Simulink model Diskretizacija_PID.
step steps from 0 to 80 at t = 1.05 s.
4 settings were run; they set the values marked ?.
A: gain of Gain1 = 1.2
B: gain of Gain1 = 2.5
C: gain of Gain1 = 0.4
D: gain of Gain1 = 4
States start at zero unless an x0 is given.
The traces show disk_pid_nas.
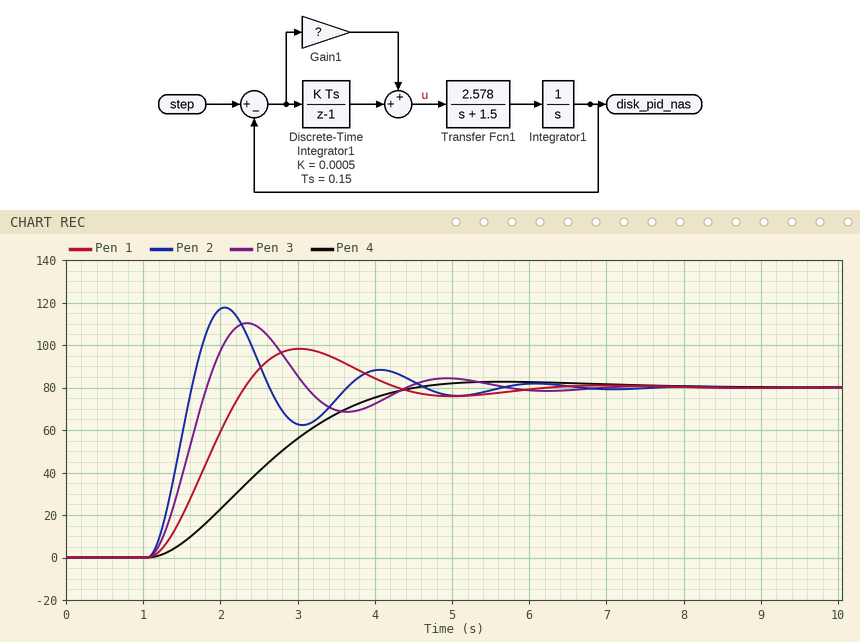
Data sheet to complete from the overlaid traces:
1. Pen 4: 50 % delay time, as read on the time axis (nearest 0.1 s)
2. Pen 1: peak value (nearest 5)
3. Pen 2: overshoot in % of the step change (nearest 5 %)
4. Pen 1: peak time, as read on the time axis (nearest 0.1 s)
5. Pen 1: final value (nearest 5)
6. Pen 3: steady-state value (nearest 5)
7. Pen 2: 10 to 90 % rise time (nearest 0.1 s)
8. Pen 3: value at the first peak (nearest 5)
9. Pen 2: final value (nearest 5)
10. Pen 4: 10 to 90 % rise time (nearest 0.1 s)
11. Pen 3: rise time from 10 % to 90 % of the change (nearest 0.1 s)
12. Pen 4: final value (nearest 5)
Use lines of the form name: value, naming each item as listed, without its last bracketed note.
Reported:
Pen 4: 50 % delay time, as read on the time axis: 2.5 s
Pen 1: peak value: 100
Pen 2: overshoot in % of the step change: 45 %
Pen 1: peak time, as read on the time axis: 3.0 s
Pen 1: final value: 80
Pen 3: steady-state value: 80
Pen 2: 10 to 90 % rise time: 0.4 s
Pen 3: value at the first peak: 110
Pen 2: final value: 80
Pen 4: 10 to 90 % rise time: 2.2 s
Pen 3: rise time from 10 % to 90 % of the change: 0.5 s
Pen 4: final value: 80
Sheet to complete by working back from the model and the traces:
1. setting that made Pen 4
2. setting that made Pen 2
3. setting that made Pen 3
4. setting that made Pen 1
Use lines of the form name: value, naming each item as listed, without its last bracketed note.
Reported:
setting that made Pen 4: C
setting that made Pen 2: D
setting that made Pen 3: B
setting that made Pen 1: A
